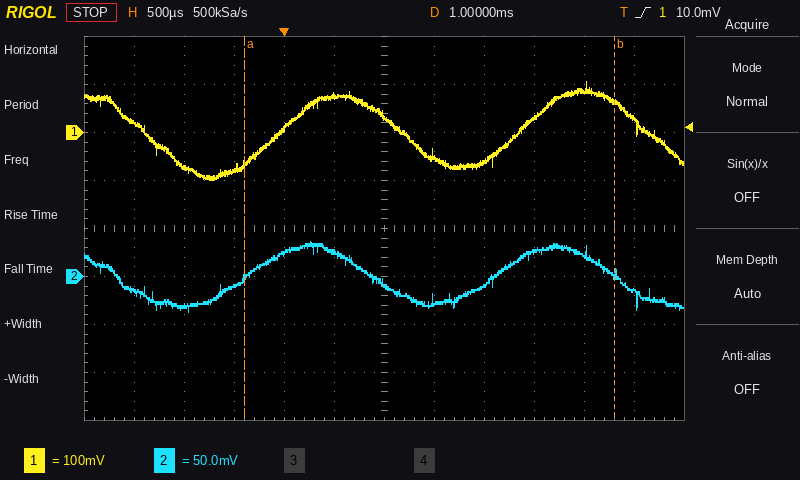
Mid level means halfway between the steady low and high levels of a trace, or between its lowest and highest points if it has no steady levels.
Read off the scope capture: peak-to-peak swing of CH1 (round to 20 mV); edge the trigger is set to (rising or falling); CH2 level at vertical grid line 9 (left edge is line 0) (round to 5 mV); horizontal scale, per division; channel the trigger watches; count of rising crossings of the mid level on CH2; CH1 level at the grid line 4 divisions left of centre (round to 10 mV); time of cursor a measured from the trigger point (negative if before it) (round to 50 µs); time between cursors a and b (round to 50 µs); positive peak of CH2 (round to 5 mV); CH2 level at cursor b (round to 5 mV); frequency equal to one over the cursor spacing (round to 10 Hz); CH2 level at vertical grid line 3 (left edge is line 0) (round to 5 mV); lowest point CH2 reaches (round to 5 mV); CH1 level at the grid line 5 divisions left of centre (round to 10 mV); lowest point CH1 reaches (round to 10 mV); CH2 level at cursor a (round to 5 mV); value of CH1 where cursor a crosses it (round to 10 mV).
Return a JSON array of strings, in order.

["200 mV", "rising", "25 mV", "500 µs", "CH1", "2", "-70 mV", "-400 µs", "3.70 ms", "35 mV", "5 mV", "270 Hz", "-10 mV", "-35 mV", "20 mV", "-100 mV", "0 mV", "-70 mV"]
